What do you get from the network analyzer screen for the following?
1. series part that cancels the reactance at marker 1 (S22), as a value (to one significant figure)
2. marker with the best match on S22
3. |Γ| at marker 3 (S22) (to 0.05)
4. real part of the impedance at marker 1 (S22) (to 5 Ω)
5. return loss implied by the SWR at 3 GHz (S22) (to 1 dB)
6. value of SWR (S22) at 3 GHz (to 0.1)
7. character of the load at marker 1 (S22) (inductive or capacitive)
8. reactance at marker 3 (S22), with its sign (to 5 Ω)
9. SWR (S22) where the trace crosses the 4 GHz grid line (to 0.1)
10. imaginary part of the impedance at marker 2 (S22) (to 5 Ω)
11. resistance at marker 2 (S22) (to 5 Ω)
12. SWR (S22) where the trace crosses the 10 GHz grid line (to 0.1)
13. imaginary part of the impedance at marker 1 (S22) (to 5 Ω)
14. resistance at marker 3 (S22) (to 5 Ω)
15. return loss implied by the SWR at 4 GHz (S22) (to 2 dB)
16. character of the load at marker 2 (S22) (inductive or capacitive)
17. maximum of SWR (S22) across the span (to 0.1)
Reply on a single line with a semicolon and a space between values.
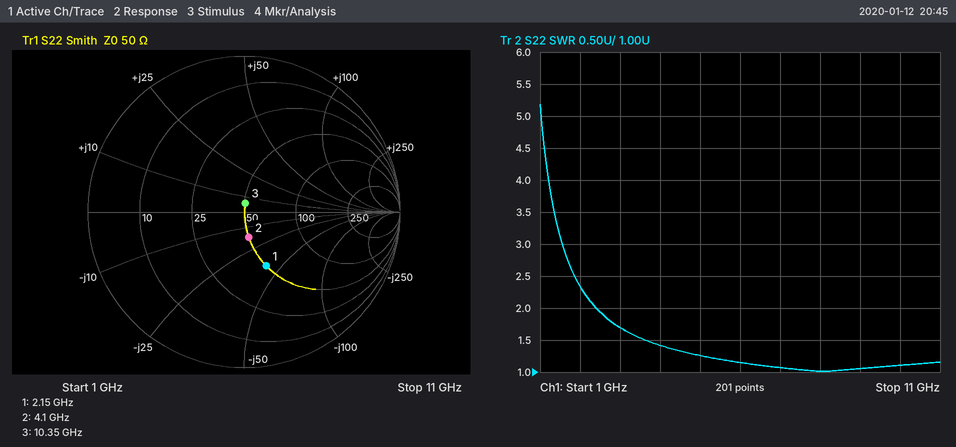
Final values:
3 nH; marker 3; 0.05; 50 Ω; 12 dB; 1.7; capacitive; +5 Ω; 1.4; -15 Ω; 50 Ω; 1.1; -40 Ω; 50 Ω; 16 dB; capacitive; 5.2
